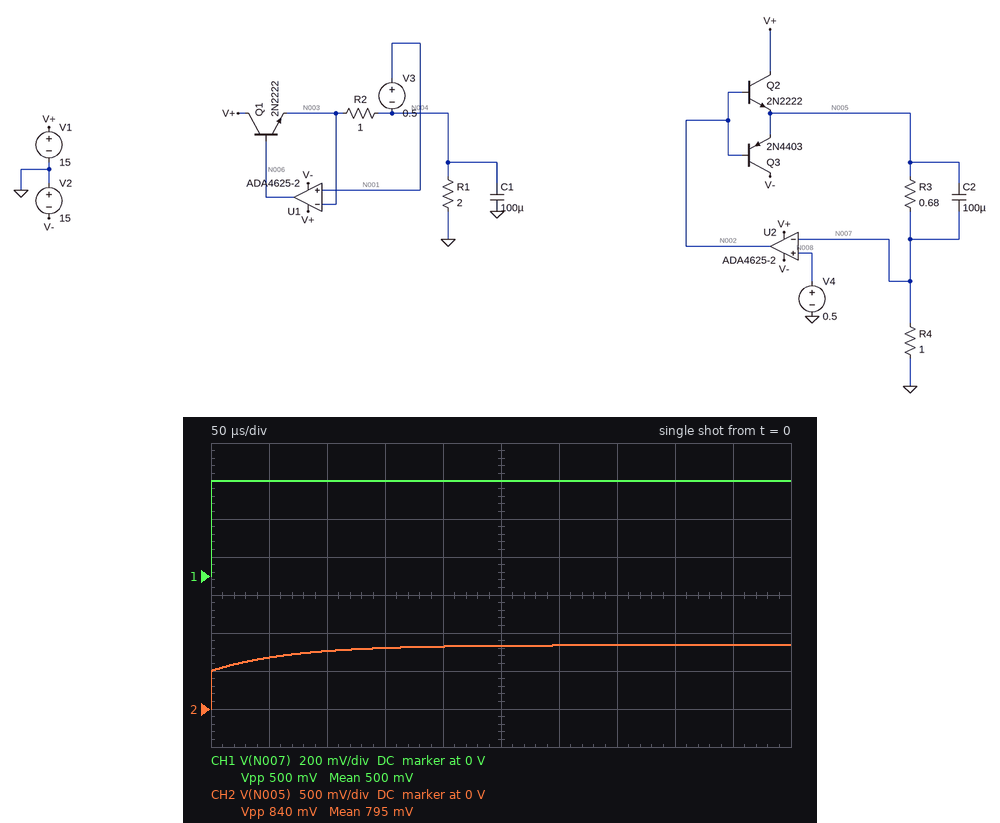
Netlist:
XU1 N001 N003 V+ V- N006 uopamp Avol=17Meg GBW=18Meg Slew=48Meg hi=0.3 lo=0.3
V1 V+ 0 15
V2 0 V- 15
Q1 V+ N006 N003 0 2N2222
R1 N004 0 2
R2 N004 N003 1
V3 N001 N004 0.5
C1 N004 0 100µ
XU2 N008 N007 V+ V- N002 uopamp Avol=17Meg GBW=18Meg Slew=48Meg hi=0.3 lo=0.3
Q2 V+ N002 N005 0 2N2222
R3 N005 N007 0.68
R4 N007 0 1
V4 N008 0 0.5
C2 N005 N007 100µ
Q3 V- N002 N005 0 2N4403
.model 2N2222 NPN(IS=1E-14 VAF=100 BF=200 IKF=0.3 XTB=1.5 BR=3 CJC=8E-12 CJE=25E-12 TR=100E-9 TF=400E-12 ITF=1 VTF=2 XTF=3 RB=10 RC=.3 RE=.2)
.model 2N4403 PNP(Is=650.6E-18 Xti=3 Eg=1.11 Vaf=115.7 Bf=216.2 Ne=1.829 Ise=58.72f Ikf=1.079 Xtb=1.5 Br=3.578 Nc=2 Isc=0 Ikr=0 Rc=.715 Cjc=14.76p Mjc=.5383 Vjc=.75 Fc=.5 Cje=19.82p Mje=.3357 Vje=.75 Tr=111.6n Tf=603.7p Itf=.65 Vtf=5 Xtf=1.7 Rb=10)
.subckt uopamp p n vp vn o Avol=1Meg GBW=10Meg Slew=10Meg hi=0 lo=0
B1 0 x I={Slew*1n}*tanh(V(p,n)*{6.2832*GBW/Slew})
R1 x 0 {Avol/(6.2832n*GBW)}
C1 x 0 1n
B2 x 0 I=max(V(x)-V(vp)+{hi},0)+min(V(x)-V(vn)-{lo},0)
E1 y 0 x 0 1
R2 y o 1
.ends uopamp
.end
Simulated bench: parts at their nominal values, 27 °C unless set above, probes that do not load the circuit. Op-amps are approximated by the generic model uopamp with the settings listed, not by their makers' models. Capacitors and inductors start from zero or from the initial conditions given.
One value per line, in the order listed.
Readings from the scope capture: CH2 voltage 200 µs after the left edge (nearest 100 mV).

800 mV
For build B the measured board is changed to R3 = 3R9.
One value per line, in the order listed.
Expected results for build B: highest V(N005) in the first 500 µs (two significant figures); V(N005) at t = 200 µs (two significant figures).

1.9 V
1.3 V
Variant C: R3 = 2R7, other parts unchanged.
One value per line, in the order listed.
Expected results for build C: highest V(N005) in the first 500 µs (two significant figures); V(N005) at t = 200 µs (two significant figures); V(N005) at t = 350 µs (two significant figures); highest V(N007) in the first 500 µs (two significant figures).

1.6 V
1.2 V
1.5 V
500 mV
